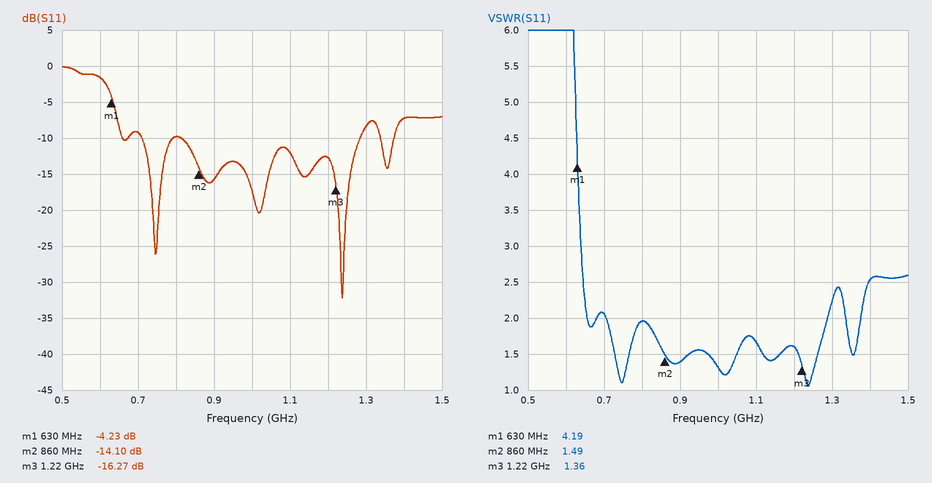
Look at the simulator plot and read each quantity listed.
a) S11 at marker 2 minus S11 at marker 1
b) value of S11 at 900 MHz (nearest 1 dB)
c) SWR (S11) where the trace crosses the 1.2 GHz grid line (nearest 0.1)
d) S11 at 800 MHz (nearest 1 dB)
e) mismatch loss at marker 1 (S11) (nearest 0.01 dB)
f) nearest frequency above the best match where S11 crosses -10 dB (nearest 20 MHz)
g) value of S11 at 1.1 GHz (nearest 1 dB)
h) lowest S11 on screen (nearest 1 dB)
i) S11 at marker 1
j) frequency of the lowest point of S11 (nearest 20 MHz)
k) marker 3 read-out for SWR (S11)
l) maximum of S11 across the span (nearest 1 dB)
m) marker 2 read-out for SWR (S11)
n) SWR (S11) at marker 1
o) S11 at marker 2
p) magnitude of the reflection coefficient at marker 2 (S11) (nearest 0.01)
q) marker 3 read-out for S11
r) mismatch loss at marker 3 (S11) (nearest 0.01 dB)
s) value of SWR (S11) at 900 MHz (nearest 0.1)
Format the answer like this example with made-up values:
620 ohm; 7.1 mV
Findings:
-9.87 dB; -16 dB; 1.6; -10 dB; 2.06 dB; 1.28 GHz; -12 dB; -32 dB; -4.23 dB; 1.24 GHz; 1.36; 0 dB; 1.49; 4.19; -14.10 dB; 0.20; -16.27 dB; 0.10 dB; 1.4
